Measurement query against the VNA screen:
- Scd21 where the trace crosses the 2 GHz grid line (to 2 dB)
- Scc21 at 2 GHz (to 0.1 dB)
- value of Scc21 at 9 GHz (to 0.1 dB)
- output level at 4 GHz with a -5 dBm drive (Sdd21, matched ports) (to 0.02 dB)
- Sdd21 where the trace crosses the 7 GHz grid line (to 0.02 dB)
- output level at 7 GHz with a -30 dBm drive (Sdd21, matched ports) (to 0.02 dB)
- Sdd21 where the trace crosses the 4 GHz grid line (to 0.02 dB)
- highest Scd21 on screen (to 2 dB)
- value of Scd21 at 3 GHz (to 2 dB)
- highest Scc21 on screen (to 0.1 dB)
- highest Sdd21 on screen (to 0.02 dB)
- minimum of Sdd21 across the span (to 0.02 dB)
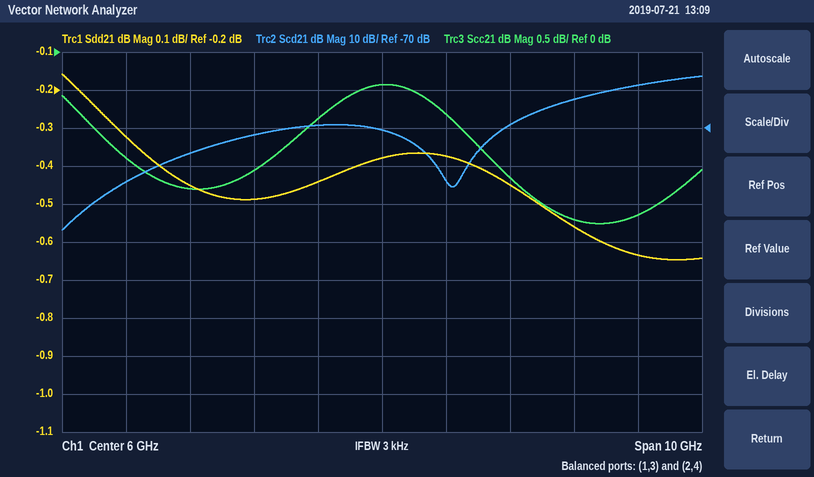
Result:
-84 dB
-1.4 dB
-2.2 dB
-5.48 dBm
-0.38 dB
-30.38 dBm
-0.48 dB
-56 dB
-76 dB
-0.4 dB
-0.16 dB
-0.64 dB
